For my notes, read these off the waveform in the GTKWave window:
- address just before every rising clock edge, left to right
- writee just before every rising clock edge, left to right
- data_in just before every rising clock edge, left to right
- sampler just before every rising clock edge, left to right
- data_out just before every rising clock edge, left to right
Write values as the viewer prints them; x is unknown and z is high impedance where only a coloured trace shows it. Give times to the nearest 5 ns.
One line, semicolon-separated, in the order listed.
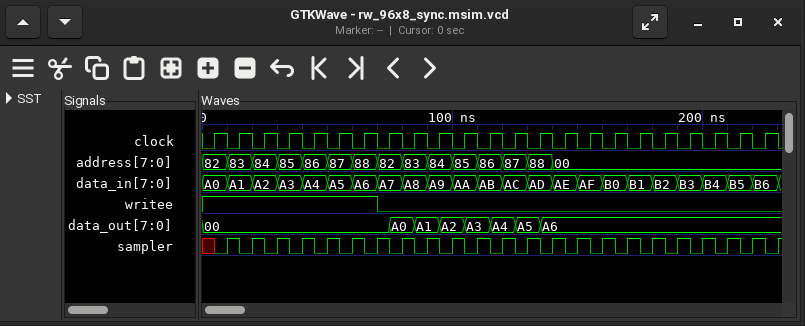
82, 83, 84, 85, 86, 87, 88, 82, 83, 84, 85, 86, 87, 88, 00, 00, 00, 00, 00, 00, 00, 00, 00; 1 1 1 1 1 1 1 0 0 0 0 0 0 0 0 0 0 0 0 0 0 0 0; A0, A1, A2, A3, A4, A5, A6, A7, A8, A9, AA, AB, AC, AD, AE, AF, B0, B1, B2, B3, B4, B5, B6; x 1 1 1 1 1 1 1 1 1 1 1 1 1 1 1 1 1 1 1 1 1 1; 00, 00, 00, 00, 00, 00, 00, 00, A0, A1, A2, A3, A4, A5, A6, A6, A6, A6, A6, A6, A6, A6, A6
